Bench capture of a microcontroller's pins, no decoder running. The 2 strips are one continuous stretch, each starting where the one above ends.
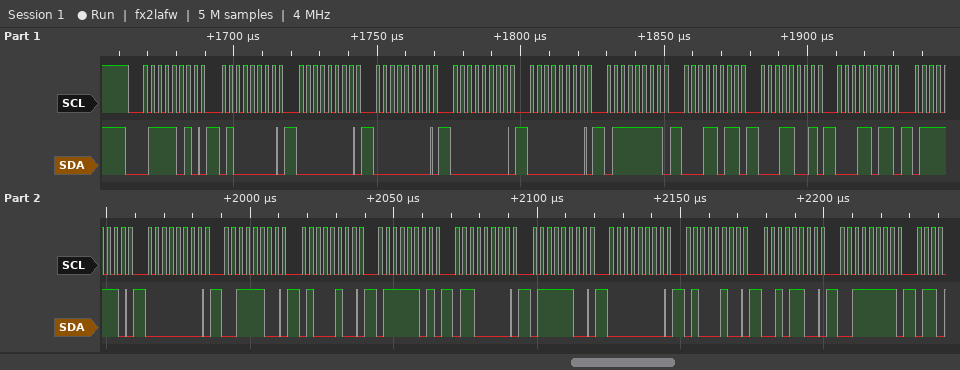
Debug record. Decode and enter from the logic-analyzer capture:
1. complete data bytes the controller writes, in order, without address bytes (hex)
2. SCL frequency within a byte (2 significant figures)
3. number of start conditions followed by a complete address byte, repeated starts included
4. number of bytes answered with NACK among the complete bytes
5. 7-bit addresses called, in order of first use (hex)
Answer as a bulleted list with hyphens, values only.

- 40 00 00 00 00 7F 1B 19 1B 7E 00 3C 44 7D 60 7C 00 44 2C 3F
- 400 kHz
- 1
- 0
- 0x3D
